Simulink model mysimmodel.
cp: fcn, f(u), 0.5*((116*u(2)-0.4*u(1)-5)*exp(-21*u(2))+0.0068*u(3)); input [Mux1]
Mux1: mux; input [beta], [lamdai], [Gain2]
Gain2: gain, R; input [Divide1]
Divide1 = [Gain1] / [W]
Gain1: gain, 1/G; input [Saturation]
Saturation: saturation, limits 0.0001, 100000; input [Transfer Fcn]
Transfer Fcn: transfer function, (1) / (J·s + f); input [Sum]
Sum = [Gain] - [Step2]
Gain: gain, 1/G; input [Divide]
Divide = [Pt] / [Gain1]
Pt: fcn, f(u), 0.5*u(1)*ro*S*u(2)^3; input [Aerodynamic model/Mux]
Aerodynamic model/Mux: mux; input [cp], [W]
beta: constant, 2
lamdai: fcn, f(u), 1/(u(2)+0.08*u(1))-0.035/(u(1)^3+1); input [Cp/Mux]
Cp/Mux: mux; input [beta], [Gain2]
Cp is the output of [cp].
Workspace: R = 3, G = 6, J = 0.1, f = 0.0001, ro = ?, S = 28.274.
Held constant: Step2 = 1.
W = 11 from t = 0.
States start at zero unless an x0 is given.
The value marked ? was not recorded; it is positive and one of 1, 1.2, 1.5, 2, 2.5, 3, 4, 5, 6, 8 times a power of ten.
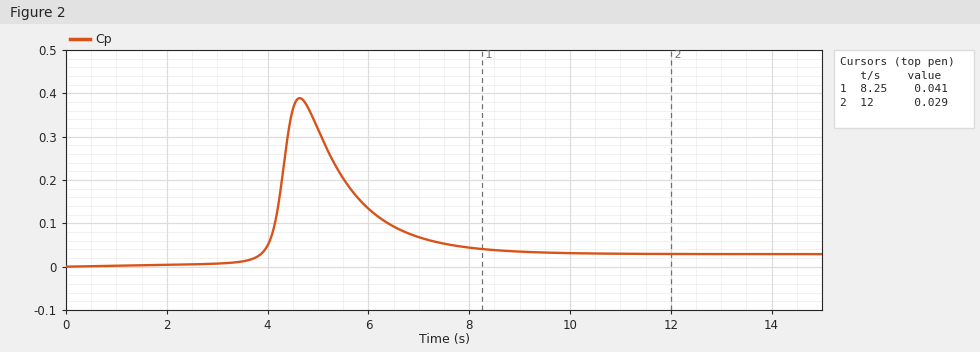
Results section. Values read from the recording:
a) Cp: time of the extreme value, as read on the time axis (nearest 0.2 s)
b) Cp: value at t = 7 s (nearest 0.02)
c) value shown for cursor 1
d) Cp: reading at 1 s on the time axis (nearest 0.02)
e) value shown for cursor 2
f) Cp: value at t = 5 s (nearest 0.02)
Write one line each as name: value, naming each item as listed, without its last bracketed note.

Cp: time of the extreme value, as read on the time axis: 4.6 s
Cp: value at t = 7 s: 0.06
value shown for cursor 1: 0.041
Cp: reading at 1 s on the time axis: 0.00
value shown for cursor 2: 0.029
Cp: value at t = 5 s: 0.32
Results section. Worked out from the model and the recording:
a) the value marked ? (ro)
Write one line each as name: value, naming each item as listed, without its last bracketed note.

the value marked ?: 0.8
